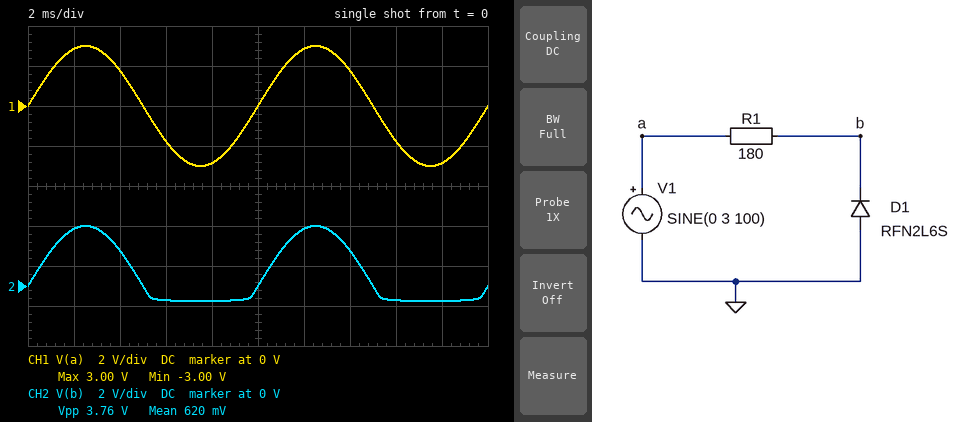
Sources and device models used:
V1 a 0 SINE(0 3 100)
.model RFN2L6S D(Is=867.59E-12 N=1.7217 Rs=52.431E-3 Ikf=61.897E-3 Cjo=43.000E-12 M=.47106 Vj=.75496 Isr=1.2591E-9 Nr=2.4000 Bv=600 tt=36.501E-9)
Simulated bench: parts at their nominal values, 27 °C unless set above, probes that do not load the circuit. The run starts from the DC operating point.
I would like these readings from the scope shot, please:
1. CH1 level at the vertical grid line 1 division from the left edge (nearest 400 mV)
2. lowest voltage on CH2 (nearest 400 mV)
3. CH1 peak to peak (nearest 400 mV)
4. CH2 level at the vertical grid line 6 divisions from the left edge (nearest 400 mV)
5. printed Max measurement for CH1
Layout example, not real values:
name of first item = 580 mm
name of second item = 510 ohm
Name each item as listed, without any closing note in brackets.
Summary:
CH1 level at the vertical grid line 1 division from the left edge = 2.8 V
lowest voltage on CH2 = -800 mV
CH1 peak to peak = 6.0 V
CH2 level at the vertical grid line 6 divisions from the left edge = 2.8 V
printed Max measurement for CH1 = 3.00 V
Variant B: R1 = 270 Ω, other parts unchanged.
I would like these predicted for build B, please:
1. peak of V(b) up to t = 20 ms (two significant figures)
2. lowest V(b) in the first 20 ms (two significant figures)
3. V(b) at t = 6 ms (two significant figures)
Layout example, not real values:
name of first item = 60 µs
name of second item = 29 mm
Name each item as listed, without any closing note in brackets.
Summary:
peak of V(b) up to t = 20 ms = 3.0 V
lowest V(b) in the first 20 ms = -730 mV
V(b) at t = 6 ms = -690 mV
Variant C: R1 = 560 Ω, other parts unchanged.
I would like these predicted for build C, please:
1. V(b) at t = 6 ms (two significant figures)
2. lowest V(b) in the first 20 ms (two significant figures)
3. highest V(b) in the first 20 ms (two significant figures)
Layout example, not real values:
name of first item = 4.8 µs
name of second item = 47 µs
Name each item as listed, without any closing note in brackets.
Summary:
V(b) at t = 6 ms = -660 mV
lowest V(b) in the first 20 ms = -700 mV
highest V(b) in the first 20 ms = 3.0 V
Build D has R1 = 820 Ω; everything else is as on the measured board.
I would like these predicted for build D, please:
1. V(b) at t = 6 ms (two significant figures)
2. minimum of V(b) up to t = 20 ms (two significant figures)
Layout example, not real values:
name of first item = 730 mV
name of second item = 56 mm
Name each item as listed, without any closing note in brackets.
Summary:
V(b) at t = 6 ms = -640 mV
minimum of V(b) up to t = 20 ms = -680 mV
